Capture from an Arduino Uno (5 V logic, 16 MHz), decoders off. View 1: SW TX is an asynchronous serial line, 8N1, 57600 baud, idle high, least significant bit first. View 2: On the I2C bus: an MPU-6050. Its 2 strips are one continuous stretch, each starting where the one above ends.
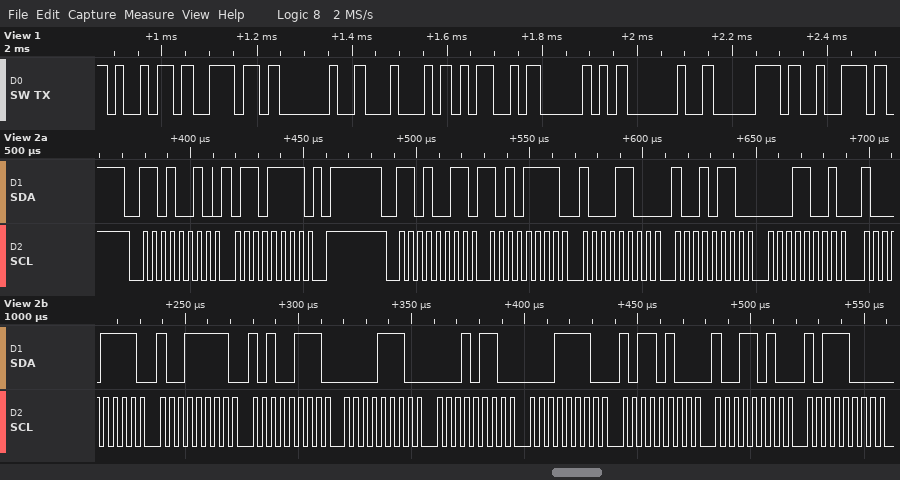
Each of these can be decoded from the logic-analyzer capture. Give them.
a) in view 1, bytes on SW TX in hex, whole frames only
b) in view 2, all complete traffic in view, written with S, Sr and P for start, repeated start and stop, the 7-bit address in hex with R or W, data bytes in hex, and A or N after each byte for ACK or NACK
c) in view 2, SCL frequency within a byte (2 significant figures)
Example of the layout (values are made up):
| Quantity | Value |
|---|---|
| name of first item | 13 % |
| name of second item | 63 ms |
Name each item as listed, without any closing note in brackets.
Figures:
| Quantity | Value |
|---|---|
| in view 1, bytes on SW TX in hex, whole frames only | 69 6E 20 44 4D 50 20 70 72 |
| in view 2, all complete traffic in view, written with S, Sr and P for start, repeated start and stop, the 7-bit address in hex with R or W, data bytes in hex, and A or N after each byte for ACK or NACK | S 69W A 6F A P S 69R A AF A 8C A 96 A 19 A 8F A 9F A A7 A 0E A 16 A 1E A B4 A 9A A B8 A |
| in view 2, SCL frequency within a byte | 250 kHz |
